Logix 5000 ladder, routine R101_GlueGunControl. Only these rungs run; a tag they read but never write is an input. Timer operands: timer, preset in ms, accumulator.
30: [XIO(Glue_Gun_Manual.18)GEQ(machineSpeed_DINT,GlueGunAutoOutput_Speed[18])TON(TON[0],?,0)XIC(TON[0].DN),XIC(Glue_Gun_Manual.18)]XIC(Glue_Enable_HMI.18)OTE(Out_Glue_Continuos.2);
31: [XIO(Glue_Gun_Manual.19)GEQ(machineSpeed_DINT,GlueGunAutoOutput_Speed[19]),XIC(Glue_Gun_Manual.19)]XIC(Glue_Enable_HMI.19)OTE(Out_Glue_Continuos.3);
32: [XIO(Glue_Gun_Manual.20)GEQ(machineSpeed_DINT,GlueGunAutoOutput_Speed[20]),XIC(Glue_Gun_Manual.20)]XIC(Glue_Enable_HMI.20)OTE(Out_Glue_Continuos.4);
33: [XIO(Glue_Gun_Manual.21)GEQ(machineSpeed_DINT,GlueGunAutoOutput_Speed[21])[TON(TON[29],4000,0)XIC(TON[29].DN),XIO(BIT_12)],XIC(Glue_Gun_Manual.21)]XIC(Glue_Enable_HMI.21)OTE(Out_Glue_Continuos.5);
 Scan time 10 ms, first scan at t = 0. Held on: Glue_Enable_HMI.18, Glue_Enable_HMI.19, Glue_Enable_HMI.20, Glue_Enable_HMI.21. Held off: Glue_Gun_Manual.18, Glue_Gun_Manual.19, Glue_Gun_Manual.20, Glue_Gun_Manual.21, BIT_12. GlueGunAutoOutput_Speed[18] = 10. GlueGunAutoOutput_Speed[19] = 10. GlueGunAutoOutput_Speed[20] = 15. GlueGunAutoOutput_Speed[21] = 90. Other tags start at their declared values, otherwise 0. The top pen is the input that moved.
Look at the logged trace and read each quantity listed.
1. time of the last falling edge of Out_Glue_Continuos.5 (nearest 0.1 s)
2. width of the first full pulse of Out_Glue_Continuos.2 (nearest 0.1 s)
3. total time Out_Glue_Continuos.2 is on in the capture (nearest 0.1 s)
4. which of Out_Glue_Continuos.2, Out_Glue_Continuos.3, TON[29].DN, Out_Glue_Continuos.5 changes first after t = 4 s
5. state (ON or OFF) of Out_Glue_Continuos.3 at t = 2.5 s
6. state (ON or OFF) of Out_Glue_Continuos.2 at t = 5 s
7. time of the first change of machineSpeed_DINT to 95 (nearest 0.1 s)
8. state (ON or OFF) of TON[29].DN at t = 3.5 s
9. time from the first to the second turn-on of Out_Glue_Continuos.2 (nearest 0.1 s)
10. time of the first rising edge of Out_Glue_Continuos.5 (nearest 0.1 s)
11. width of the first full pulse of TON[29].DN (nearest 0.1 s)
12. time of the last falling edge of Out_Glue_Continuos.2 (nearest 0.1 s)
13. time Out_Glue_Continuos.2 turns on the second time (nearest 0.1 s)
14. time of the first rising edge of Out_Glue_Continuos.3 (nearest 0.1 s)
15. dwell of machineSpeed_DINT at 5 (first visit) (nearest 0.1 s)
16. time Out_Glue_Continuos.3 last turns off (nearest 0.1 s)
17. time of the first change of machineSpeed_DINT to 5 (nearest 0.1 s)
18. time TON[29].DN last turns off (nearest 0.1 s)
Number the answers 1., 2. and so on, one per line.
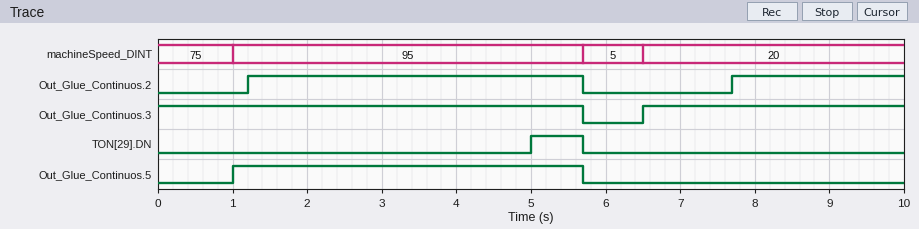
1. 5.7 s
2. 4.5 s
3. 6.8 s
4. TON[29].DN
5. ON
6. ON
7. 1.0 s
8. OFF
9. 6.5 s
10. 1.0 s
11. 0.7 s
12. 5.7 s
13. 7.7 s
14. 6.5 s
15. 0.8 s
16. 5.7 s
17. 5.7 s
18. 5.7 s
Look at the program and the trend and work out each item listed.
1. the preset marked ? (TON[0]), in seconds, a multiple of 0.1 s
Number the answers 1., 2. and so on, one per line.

1. 1.2 s
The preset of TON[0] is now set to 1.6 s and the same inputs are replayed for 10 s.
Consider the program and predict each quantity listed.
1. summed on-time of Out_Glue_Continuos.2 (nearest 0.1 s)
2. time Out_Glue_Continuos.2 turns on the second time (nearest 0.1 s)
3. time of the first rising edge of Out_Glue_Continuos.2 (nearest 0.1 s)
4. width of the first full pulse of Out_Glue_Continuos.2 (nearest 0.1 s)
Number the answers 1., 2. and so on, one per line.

1. 6.0 s
2. 8.1 s
3. 1.6 s
4. 4.1 s
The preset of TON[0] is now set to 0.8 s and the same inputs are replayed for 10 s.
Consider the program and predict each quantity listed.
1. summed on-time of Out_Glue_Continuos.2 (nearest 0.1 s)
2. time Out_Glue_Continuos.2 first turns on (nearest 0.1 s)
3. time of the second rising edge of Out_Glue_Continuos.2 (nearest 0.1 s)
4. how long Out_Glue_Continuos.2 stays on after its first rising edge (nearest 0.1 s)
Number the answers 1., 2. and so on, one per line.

1. 7.6 s
2. 0.8 s
3. 7.3 s
4. 4.9 s
